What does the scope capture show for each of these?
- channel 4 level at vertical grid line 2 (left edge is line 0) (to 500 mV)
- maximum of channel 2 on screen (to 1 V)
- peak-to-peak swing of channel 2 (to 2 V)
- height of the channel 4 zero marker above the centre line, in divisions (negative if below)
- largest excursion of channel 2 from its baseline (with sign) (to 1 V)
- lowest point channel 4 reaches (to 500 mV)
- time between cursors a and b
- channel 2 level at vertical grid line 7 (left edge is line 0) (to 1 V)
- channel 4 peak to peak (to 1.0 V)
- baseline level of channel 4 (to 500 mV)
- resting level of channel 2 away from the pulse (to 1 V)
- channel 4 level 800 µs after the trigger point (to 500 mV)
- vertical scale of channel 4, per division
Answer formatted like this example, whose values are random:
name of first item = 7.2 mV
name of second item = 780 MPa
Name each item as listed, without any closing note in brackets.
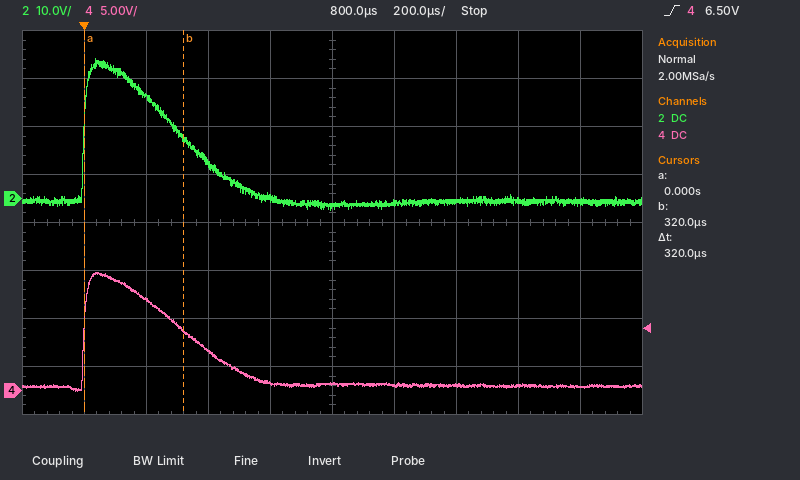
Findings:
channel 4 level at vertical grid line 2 (left edge is line 0) = 9.5 V
maximum of channel 2 on screen = 29 V
peak-to-peak swing of channel 2 = 32 V
height of the channel 4 zero marker above the centre line, in divisions = -3.5 div
largest excursion of channel 2 from its baseline (with sign) = +30 V
lowest point channel 4 reaches = 0.0 V
time between cursors a and b = 320 µs
channel 2 level at vertical grid line 7 (left edge is line 0) = -1 V
channel 4 peak to peak = 12.0 V
baseline level of channel 4 = 500 mV
resting level of channel 2 away from the pulse = -1 V
channel 4 level 800 µs after the trigger point = 500 mV
vertical scale of channel 4, per division = 5 V
